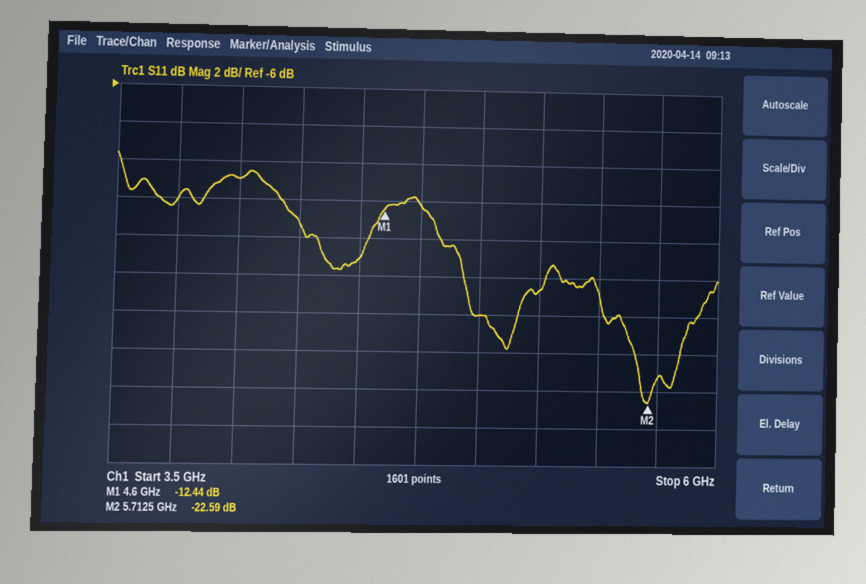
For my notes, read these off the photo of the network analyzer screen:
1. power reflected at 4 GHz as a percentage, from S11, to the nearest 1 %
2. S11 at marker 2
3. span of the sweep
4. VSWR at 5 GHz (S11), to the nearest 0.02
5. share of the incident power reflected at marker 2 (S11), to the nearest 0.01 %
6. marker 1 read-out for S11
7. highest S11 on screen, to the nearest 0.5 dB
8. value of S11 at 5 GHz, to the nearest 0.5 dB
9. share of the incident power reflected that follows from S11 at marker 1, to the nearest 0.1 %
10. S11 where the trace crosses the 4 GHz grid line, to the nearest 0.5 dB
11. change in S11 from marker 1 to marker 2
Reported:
8 %
-22.59 dB
2.5 GHz
1.28
0.55 %
-12.44 dB
-9.5 dB
-18.0 dB
5.7 %
-11.0 dB
-10.15 dB
